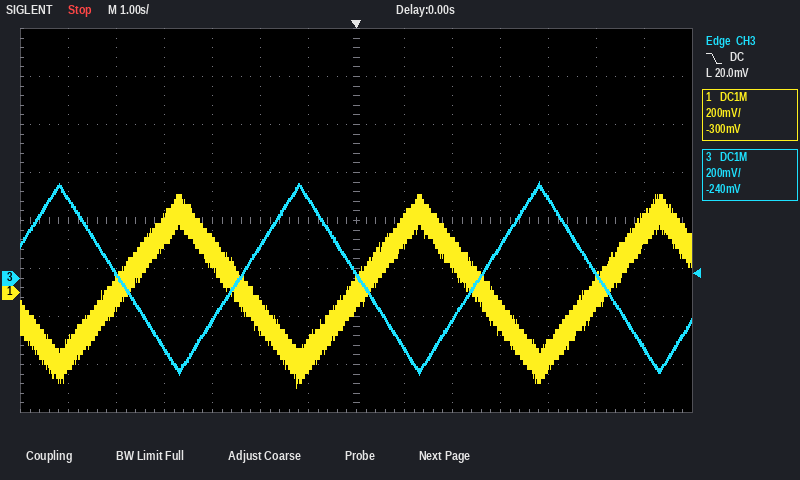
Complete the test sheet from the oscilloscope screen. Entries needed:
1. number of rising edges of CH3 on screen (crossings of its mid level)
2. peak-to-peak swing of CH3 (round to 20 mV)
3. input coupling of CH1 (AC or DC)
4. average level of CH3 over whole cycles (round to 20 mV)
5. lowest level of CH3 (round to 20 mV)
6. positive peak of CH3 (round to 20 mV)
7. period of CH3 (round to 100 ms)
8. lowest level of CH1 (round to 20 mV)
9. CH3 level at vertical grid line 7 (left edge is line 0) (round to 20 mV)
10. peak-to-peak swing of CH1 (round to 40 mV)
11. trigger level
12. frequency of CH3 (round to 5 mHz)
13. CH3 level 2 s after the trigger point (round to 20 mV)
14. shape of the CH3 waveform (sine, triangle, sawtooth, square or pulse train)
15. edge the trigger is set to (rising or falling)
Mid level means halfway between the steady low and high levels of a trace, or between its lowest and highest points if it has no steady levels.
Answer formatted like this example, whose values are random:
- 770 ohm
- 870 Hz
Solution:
- 2
- 800 mV
- DC
- 0 mV
- -400 mV
- 400 mV
- 5.0 s
- -400 mV
- 20 mV
- 800 mV
- 20.0 mV
- 200 mHz
- -180 mV
- triangle
- falling
